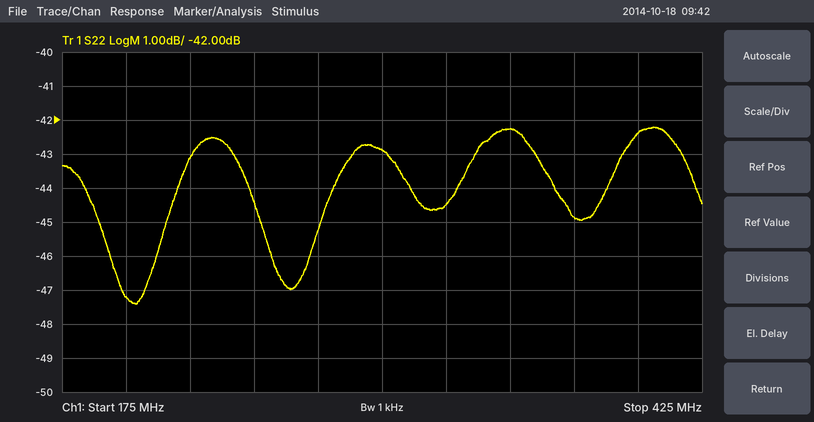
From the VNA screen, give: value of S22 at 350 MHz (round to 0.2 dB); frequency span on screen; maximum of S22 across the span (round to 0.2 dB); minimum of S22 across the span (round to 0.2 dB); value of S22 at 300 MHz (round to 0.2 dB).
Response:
-42.2 dB
250 MHz
-42.2 dB
-47.4 dB
-42.8 dB
